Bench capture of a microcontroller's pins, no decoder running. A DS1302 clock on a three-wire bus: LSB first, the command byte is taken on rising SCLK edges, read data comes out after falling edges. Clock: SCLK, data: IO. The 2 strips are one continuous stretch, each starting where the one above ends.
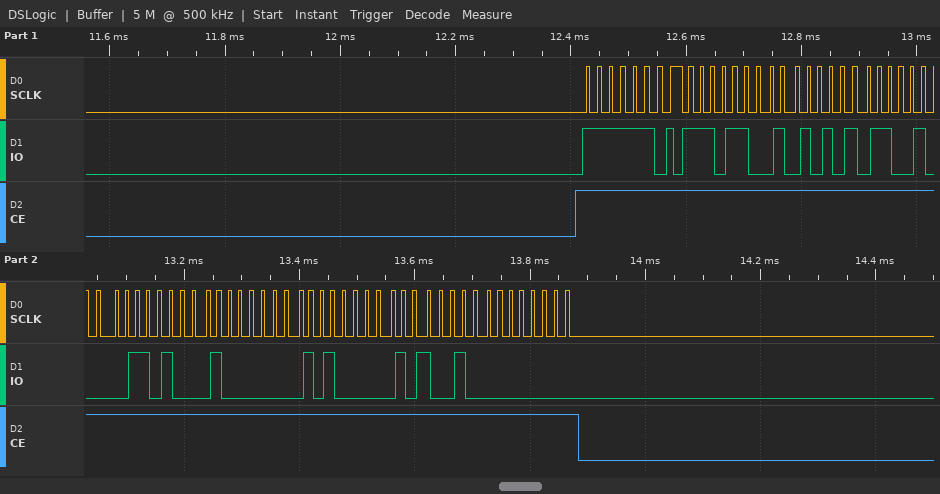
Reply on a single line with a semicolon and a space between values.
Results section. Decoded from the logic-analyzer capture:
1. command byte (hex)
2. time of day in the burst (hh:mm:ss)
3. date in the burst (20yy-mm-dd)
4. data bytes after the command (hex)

0xBF; 13:55:37; 2025-01-16; 37 55 13 16 01 05 25 00
